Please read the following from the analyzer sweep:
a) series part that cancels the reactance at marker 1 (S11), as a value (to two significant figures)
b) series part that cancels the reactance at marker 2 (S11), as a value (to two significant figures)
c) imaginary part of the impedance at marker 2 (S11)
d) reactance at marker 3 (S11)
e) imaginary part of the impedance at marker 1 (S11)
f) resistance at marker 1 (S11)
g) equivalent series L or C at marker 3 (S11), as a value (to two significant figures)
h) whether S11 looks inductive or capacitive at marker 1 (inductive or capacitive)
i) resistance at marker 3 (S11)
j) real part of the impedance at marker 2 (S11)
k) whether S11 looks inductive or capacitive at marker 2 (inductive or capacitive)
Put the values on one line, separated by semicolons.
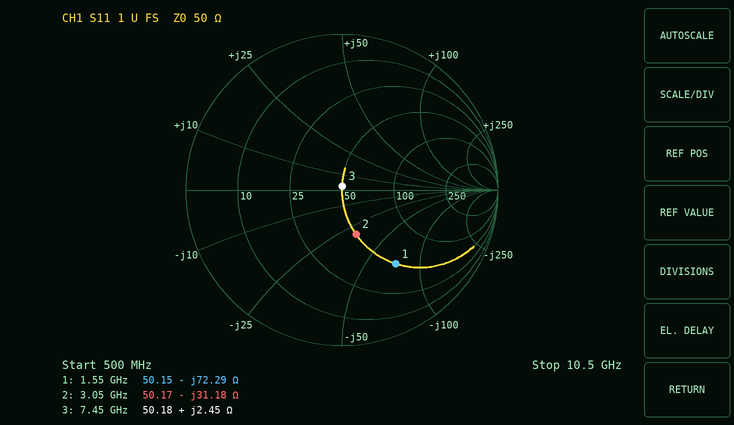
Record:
7.4 nH; 1.6 nH; -31.18 Ω; +2.45 Ω; -72.29 Ω; 50.15 Ω; 52 pH; capacitive; 50.18 Ω; 50.17 Ω; capacitive
